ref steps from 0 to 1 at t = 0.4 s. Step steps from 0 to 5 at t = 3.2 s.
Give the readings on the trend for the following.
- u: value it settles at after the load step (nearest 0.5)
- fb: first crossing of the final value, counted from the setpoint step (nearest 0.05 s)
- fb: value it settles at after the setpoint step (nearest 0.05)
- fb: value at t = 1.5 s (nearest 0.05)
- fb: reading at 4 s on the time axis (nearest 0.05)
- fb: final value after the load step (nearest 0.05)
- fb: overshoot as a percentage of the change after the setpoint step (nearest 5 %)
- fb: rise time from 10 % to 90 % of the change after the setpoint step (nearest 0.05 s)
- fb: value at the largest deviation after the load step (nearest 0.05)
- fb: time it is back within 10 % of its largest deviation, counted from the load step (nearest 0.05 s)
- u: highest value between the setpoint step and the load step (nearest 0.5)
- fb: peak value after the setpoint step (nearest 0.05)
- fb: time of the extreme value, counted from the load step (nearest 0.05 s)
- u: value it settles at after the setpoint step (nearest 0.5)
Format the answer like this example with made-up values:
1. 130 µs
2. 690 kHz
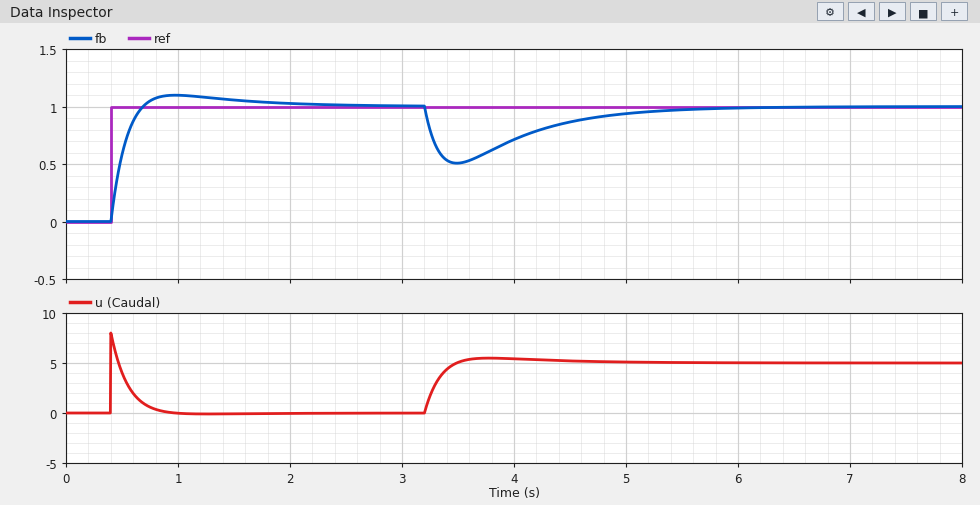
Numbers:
1. 5.0
2. 0.30 s
3. 1.00
4. 1.05
5. 0.70
6. 1.00
7. 10 %
8. 0.20 s
9. 0.50
10. 1.95 s
11. 8.0
12. 1.10
13. 0.30 s
14. 0.0
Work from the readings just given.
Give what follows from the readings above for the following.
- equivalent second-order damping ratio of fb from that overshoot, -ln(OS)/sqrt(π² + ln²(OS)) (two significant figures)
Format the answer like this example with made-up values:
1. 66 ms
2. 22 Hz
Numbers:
1. 0.59
